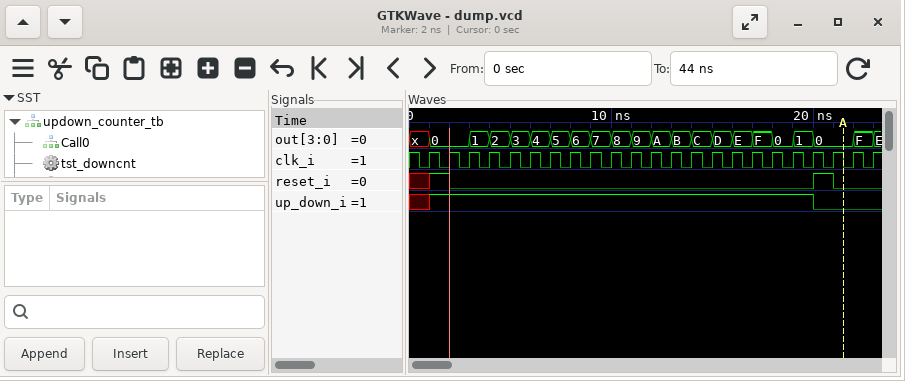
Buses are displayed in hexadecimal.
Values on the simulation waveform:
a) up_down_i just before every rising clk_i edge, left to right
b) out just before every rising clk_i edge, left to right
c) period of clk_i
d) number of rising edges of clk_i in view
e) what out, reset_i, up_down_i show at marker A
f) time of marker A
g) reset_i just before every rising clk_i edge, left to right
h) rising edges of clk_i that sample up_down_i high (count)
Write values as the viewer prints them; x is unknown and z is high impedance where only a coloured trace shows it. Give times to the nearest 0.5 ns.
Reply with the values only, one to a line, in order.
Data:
x 1 1 1 1 1 1 1 1 1 1 1 1 1 1 1 1 1 1 1 0 0 0
x, 0, 0, 1, 2, 3, 4, 5, 6, 7, 8, 9, A, B, C, D, E, F, 0, 1, 0, 0, F
1 ns
23
out=0, reset_i=0, up_down_i=0
21.5 ns
x 1 0 0 0 0 0 0 0 0 0 0 0 0 0 0 0 0 0 0 1 0 0
19
